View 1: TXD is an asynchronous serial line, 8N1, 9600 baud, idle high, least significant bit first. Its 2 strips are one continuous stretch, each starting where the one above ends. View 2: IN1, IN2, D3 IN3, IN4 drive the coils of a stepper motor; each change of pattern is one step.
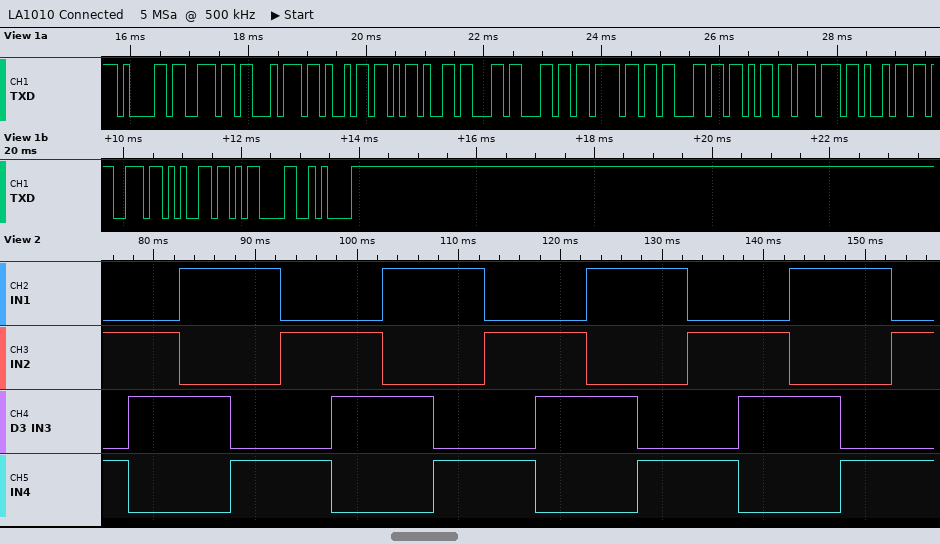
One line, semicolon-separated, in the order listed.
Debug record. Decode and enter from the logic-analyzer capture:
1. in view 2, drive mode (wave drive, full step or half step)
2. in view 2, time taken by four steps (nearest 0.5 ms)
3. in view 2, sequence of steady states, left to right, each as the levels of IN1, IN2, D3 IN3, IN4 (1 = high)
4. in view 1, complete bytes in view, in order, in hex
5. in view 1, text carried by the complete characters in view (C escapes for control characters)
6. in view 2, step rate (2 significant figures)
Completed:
full step; 20.0 ms; 0101 0110 1010 1001 0101 0110 1010 1001 0101 0110 1010 1001 0101 0110 1010 1001 0101; 0x61 0x6E 0x74 0x69 0x2D 0x63 0x6C 0x6F 0x63 0x6B 0x77 0x69 0x73 0x65 0x0D 0x0A; "anti-clockwise\r\n"; 200 steps/s
